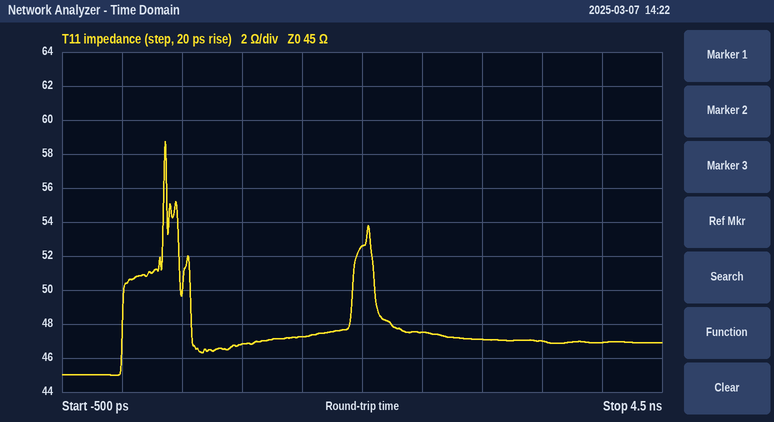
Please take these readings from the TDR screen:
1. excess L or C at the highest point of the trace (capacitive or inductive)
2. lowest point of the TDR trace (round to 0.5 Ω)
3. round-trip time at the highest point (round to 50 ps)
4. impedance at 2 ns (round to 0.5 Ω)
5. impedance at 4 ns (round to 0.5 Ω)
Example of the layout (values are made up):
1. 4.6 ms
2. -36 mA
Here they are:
1. inductive
2. 45.0 Ω
3. 350 ps
4. 52.5 Ω
5. 47.0 Ω
